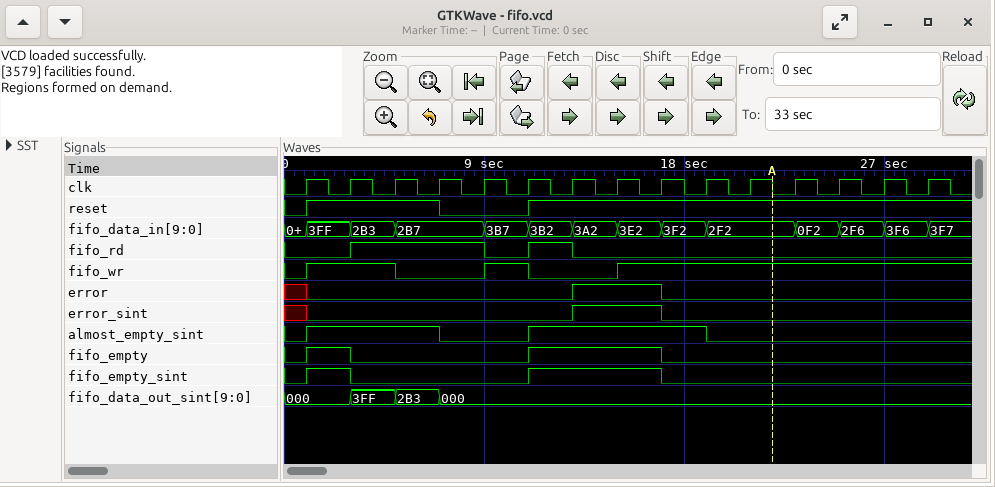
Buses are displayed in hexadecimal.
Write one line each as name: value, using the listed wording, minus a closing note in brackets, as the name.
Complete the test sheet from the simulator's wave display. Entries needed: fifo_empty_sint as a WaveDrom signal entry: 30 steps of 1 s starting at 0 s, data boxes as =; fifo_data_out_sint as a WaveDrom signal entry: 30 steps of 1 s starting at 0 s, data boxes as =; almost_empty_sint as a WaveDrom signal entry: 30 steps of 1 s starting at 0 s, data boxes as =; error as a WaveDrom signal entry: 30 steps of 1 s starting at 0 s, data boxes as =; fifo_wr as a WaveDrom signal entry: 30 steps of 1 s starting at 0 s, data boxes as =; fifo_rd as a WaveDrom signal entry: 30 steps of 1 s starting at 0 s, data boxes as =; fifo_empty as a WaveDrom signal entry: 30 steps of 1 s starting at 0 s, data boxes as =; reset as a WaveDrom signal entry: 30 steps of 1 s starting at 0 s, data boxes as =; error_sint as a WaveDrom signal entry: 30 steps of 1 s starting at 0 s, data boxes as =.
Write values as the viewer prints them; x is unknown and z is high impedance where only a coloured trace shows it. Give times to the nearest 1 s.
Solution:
fifo_empty_sint as a WaveDrom signal entry: 30 steps of 1 s starting at 0 s, data boxes as =: {name: 'fifo_empty_sint', wave: '01.0.......1.....0............'}
fifo_data_out_sint as a WaveDrom signal entry: 30 steps of 1 s starting at 0 s, data boxes as =: {name: 'fifo_data_out_sint', wave: '=..=.=.=......................', data: '000 3FF 2B3 000'}
almost_empty_sint as a WaveDrom signal entry: 30 steps of 1 s starting at 0 s, data boxes as =: {name: 'almost_empty_sint', wave: '01.....0...1.......0..........'}
error as a WaveDrom signal entry: 30 steps of 1 s starting at 0 s, data boxes as =: {name: 'error', wave: 'x0...........1...0............'}
fifo_wr as a WaveDrom signal entry: 30 steps of 1 s starting at 0 s, data boxes as =: {name: 'fifo_wr', wave: '01...0...1.0...1..............'}
fifo_rd as a WaveDrom signal entry: 30 steps of 1 s starting at 0 s, data boxes as =: {name: 'fifo_rd', wave: '0..1.....0.1.0................'}
fifo_empty as a WaveDrom signal entry: 30 steps of 1 s starting at 0 s, data boxes as =: {name: 'fifo_empty', wave: '01.0.......1.....0............'}
reset as a WaveDrom signal entry: 30 steps of 1 s starting at 0 s, data boxes as =: {name: 'reset', wave: '01.....0...1..................'}
error_sint as a WaveDrom signal entry: 30 steps of 1 s starting at 0 s, data boxes as =: {name: 'error_sint', wave: 'x0...........1...0............'}
